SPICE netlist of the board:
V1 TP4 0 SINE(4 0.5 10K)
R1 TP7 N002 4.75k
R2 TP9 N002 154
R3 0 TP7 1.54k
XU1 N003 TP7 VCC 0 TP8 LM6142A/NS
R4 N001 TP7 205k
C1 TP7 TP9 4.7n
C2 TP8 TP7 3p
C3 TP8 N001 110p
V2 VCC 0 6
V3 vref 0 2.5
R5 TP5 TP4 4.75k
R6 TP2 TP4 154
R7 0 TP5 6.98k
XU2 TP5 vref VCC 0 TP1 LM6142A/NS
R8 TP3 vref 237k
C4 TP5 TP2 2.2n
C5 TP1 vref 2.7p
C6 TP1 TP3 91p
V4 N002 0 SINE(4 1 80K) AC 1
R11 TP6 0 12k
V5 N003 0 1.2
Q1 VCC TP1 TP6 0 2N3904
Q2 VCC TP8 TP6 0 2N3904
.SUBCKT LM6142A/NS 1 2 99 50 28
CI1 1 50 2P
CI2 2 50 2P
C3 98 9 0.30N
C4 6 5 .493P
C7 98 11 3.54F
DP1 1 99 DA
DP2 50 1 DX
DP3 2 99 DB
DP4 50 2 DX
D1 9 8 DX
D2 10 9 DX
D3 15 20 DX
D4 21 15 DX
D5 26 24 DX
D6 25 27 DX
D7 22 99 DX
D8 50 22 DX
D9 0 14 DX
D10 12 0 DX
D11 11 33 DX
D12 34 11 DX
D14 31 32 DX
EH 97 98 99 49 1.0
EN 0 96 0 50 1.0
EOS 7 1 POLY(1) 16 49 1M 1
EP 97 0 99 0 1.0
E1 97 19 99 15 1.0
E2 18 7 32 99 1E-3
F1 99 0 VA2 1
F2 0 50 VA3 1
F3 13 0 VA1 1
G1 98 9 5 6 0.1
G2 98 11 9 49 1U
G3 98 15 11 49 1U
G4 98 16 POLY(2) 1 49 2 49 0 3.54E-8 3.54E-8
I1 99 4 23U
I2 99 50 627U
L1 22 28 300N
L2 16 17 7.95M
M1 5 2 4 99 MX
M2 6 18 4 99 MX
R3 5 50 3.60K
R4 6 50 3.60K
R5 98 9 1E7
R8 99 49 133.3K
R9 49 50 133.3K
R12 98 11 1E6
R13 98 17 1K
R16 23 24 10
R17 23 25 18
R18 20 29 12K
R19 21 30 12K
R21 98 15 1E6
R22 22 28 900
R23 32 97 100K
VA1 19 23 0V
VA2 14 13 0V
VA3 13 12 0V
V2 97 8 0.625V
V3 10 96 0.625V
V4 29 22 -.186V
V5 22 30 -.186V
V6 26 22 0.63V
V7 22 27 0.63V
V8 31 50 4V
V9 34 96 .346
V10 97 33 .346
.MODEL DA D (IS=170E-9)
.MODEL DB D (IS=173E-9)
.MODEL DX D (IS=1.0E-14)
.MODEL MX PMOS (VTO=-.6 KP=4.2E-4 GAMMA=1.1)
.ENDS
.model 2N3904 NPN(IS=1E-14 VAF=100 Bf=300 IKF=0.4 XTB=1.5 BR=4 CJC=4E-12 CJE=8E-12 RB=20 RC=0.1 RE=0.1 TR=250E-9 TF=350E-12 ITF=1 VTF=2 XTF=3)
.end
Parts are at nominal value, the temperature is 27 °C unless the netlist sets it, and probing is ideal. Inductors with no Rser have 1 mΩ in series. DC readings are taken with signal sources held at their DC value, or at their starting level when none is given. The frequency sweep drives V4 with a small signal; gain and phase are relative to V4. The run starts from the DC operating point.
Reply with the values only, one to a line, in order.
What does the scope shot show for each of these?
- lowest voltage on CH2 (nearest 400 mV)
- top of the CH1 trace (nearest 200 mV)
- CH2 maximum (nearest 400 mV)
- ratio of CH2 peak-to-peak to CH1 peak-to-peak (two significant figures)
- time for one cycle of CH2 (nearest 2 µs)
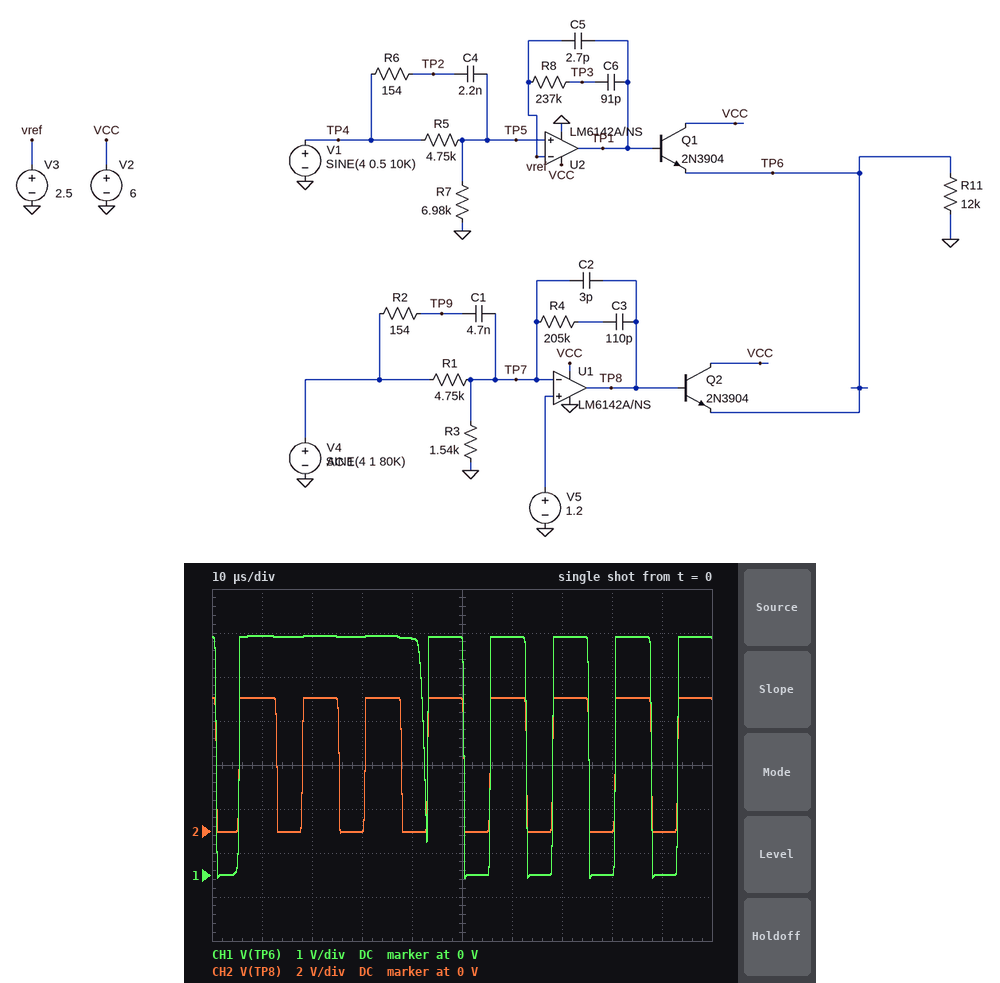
0 V
5.4 V
6.0 V
1.1
12 µs
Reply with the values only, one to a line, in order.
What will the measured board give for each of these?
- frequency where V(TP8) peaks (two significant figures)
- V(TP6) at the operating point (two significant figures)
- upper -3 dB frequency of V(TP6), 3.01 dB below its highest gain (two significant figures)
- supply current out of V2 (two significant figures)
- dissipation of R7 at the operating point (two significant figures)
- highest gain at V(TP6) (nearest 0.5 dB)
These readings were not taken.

90 MHz
5.4 V
190 MHz
1.8 mA
810 µW
-6.5 dB
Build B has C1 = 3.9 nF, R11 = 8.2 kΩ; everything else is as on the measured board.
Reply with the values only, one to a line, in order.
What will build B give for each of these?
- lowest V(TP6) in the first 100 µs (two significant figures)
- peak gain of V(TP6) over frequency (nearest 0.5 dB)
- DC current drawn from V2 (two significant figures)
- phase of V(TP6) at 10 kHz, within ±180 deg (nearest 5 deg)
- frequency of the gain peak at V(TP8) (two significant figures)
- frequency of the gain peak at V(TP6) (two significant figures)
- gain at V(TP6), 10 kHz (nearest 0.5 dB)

-140 mV
-6.0 dB
2.0 mA
-150 deg
92 MHz
91 MHz
-38.0 dB
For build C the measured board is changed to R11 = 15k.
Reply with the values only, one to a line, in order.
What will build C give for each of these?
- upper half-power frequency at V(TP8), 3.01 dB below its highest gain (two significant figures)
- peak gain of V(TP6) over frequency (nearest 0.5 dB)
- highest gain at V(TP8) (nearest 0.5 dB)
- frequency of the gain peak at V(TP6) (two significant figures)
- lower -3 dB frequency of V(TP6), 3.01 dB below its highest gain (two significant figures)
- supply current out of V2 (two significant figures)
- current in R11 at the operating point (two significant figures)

190 MHz
-7.0 dB
-6.0 dB
130 MHz
73 MHz
1.7 mA
360 µA
